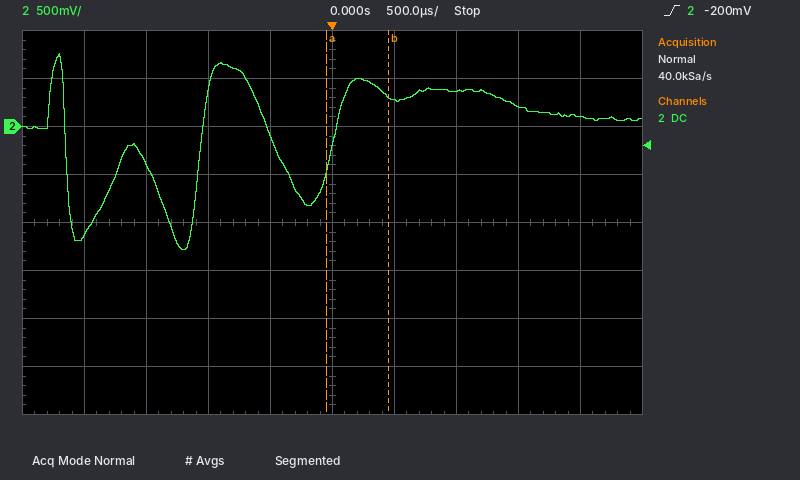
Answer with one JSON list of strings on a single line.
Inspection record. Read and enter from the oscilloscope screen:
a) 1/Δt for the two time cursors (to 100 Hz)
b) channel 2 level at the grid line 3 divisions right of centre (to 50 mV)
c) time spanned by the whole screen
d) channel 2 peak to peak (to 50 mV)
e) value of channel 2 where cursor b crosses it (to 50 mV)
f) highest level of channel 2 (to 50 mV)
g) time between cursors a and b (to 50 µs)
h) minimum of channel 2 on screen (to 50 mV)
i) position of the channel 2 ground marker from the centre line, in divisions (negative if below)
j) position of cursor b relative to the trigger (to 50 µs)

["2.0 kHz", "200 mV", "5 ms", "2.05 V", "300 mV", "750 mV", "500 µs", "-1.30 V", "+2.0 div", "+450 µs"]
